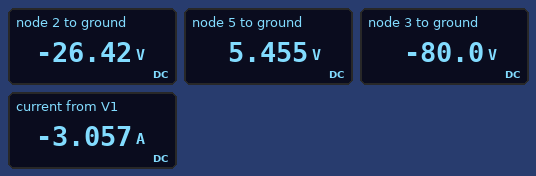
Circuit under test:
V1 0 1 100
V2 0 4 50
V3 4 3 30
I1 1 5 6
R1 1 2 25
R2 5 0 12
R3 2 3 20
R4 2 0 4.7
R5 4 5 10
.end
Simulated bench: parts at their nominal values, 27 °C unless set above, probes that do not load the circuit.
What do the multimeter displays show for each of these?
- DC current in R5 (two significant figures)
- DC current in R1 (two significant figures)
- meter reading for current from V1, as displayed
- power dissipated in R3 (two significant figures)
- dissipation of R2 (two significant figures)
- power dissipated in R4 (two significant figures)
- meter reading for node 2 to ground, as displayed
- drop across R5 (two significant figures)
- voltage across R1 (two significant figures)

5.5 A
2.9 A
-3.057 A
140 W
2.5 W
150 W
-26.42 V
55 V
74 V
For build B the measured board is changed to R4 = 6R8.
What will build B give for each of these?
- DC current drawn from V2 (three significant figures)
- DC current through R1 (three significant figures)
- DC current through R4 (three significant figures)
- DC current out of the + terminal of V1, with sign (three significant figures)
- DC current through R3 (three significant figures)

7.86 A
2.65 A
4.96 A
-3.35 A
2.31 A
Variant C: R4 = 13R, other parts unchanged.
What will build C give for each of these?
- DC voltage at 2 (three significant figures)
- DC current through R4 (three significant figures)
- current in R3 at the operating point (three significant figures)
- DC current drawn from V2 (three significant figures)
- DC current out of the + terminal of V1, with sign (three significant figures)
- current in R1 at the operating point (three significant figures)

-47.9 V
3.69 A
1.60 A
7.15 A
-3.92 A
2.08 A
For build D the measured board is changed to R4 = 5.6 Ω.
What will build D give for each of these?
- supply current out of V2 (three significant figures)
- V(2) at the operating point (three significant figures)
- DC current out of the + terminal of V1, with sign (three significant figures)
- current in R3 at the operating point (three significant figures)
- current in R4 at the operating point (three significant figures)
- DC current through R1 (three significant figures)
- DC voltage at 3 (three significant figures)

8.06 A
-29.8 V
-3.19 A
2.51 A
5.32 A
2.81 A
-80.0 V
